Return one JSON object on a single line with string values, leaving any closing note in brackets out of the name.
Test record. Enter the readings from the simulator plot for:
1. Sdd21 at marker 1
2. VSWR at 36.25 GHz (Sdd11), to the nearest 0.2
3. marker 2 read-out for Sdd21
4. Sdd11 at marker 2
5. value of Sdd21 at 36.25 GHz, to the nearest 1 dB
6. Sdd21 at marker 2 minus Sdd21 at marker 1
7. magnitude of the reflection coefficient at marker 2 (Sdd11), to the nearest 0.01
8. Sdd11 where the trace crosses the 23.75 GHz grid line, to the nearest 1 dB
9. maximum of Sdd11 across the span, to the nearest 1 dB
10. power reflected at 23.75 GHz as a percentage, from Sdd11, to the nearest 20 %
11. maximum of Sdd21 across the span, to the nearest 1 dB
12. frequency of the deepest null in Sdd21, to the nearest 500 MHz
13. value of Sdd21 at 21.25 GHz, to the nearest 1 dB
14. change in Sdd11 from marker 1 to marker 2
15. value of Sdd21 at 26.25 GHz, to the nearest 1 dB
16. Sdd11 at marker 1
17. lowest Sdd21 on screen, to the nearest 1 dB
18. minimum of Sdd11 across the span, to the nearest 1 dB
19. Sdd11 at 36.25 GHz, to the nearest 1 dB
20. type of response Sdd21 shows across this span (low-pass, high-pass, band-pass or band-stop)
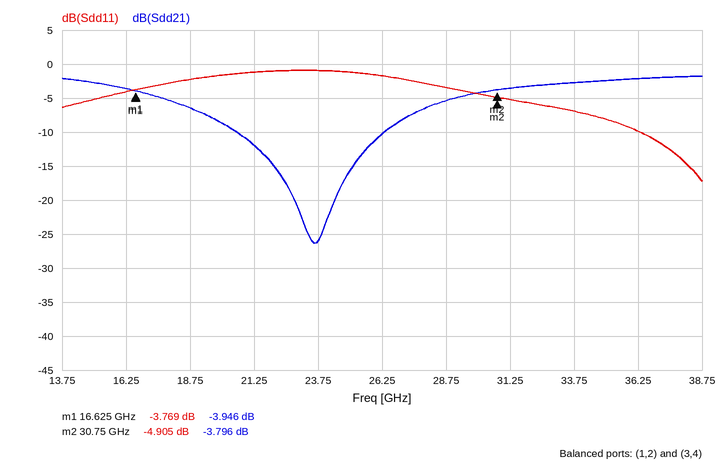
{"Sdd21 at marker 1": "-3.946 dB", "VSWR at 36.25 GHz (Sdd11), to the nearest 0.2": "2.0", "marker 2 read-out for Sdd21": "-3.796 dB", "Sdd11 at marker 2": "-4.905 dB", "value of Sdd21 at 36.25 GHz, to the nearest 1 dB": "-2 dB", "Sdd21 at marker 2 minus Sdd21 at marker 1": "0.150 dB", "magnitude of the reflection coefficient at marker 2 (Sdd11), to the nearest 0.01": "0.57", "Sdd11 where the trace crosses the 23.75 GHz grid line, to the nearest 1 dB": "-1 dB", "maximum of Sdd11 across the span, to the nearest 1 dB": "-1 dB", "power reflected at 23.75 GHz as a percentage, from Sdd11, to the nearest 20 %": "80 %", "maximum of Sdd21 across the span, to the nearest 1 dB": "-2 dB", "frequency of the deepest null in Sdd21, to the nearest 500 MHz": "23.5 GHz", "value of Sdd21 at 21.25 GHz, to the nearest 1 dB": "-12 dB", "change in Sdd11 from marker 1 to marker 2": "-1.136 dB", "value of Sdd21 at 26.25 GHz, to the nearest 1 dB": "-10 dB", "Sdd11 at marker 1": "-3.769 dB", "lowest Sdd21 on screen, to the nearest 1 dB": "-26 dB", "minimum of Sdd11 across the span, to the nearest 1 dB": "-17 dB", "Sdd11 at 36.25 GHz, to the nearest 1 dB": "-10 dB", "type of response Sdd21 shows across this span": "band-stop"}
